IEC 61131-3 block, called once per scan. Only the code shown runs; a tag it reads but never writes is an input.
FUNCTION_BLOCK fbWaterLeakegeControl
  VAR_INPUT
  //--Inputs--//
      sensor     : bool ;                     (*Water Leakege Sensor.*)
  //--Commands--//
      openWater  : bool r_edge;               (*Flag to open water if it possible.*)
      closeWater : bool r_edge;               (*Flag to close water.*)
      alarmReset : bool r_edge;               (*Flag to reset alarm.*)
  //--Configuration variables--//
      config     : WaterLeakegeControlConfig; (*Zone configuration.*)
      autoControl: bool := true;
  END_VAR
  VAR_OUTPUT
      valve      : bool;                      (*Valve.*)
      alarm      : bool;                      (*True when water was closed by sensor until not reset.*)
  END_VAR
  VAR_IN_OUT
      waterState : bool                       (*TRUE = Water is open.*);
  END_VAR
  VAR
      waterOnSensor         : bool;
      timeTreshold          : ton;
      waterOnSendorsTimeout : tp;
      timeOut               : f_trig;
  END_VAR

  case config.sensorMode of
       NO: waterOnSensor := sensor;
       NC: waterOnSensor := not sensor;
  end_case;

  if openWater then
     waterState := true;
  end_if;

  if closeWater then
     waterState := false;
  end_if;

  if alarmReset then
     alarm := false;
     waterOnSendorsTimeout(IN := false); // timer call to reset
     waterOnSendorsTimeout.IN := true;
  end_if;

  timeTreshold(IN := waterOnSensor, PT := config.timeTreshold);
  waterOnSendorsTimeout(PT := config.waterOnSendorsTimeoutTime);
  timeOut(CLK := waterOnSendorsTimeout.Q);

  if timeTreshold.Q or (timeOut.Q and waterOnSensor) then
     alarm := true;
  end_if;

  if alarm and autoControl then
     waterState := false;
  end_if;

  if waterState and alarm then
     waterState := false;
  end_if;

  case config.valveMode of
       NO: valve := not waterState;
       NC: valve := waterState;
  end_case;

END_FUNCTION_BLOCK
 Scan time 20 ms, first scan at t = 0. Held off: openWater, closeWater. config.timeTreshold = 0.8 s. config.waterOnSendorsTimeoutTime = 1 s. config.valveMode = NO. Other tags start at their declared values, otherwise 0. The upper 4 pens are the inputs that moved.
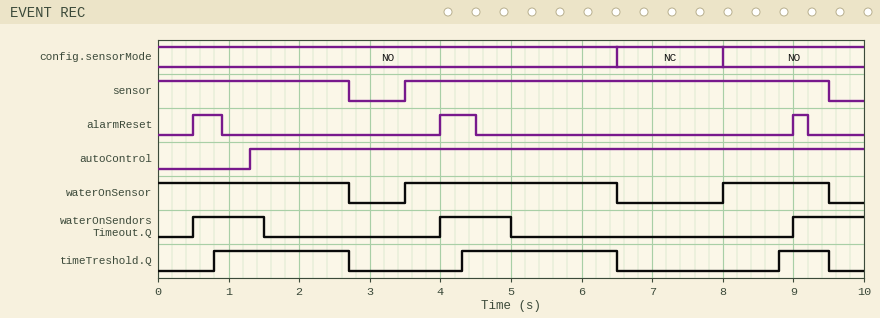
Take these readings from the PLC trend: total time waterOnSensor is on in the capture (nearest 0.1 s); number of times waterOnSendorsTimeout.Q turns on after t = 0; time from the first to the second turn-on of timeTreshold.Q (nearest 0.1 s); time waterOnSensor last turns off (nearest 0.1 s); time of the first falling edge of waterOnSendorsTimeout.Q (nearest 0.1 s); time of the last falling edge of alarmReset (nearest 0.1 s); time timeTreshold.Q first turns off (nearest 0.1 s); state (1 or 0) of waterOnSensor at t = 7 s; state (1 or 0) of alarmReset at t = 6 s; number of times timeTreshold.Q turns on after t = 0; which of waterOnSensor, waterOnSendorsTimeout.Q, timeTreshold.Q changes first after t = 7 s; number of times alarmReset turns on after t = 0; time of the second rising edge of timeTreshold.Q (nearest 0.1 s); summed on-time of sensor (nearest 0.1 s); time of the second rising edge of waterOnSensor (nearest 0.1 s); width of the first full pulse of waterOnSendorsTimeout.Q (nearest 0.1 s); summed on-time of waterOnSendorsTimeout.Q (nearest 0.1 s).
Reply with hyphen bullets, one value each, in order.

- 7.2 s
- 3
- 3.5 s
- 9.5 s
- 1.5 s
- 9.2 s
- 2.7 s
- 0
- 0
- 3
- waterOnSensor
- 3
- 4.3 s
- 8.7 s
- 8.0 s
- 1.0 s
- 3.0 s
